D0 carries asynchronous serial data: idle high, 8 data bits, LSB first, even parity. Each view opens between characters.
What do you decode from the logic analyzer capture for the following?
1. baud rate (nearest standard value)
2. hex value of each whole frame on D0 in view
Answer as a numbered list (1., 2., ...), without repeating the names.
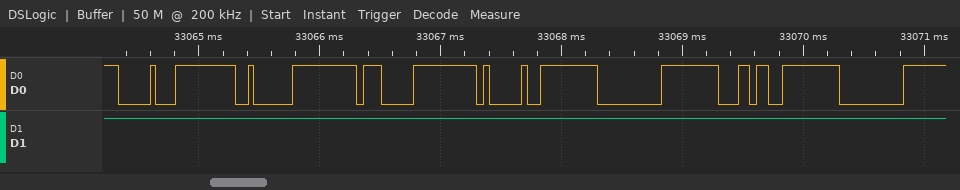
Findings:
1. 19200 baud
2. 10, 02, 07, 41, 00, 6C, 00
